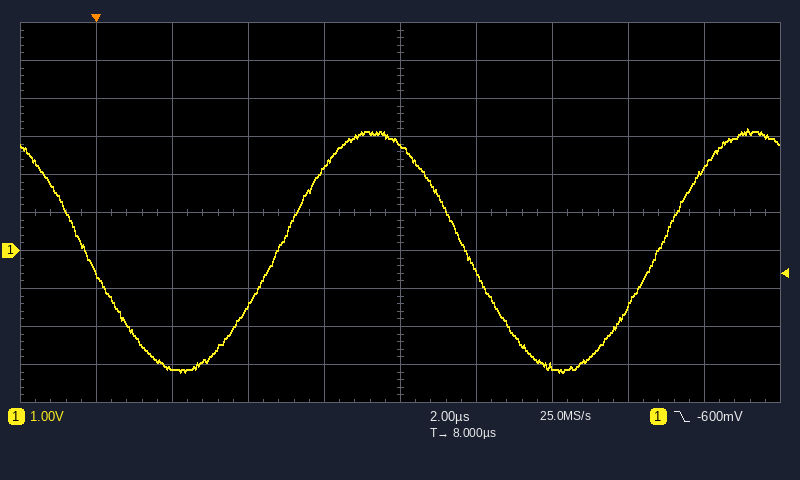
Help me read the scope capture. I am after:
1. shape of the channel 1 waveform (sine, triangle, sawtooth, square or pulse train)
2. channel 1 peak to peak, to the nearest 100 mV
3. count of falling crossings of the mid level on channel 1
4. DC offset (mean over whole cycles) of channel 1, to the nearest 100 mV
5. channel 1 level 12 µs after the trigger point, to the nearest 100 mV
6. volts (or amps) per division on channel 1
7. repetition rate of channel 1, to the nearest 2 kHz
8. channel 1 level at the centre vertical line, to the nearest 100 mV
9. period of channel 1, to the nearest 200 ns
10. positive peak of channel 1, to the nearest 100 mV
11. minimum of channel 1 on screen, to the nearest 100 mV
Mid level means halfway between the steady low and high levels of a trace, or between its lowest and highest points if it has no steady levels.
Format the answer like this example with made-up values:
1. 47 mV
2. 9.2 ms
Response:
1. sine
2. 6.4 V
3. 2
4. 0.0 V
5. -3.0 V
6. 1 V
7. 100 kHz
8. 2.8 V
9. 10.0 µs
10. 3.2 V
11. -3.2 V
